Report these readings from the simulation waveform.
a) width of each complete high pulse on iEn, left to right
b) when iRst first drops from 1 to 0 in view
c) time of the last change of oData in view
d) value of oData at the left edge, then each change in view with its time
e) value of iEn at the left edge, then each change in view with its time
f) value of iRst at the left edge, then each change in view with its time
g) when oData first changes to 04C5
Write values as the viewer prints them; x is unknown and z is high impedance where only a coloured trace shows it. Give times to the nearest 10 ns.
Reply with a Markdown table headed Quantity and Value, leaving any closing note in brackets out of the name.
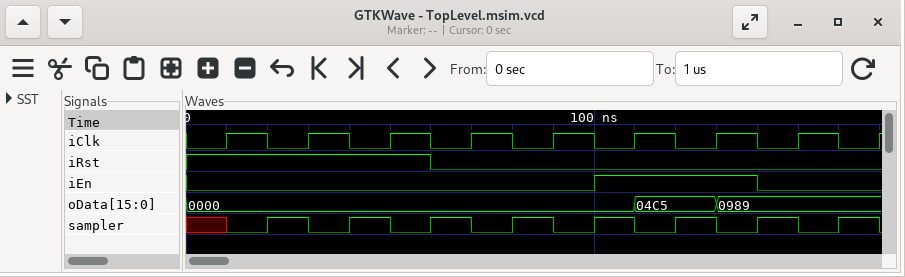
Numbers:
| Quantity | Value |
|---|---|
| width of each complete high pulse on iEn, left to right | 40 ns |
| when iRst first drops from 1 to 0 in view | 60 ns |
| time of the last change of oData in view | 130 ns |
| value of oData at the left edge, then each change in view with its time | 0000, 04C5 at 110 ns, 0989 at 130 ns |
| value of iEn at the left edge, then each change in view with its time | 0, 1 at 100 ns, 0 at 140 ns |
| value of iRst at the left edge, then each change in view with its time | 1, 0 at 60 ns |
| when oData first changes to 04C5 | 110 ns |
